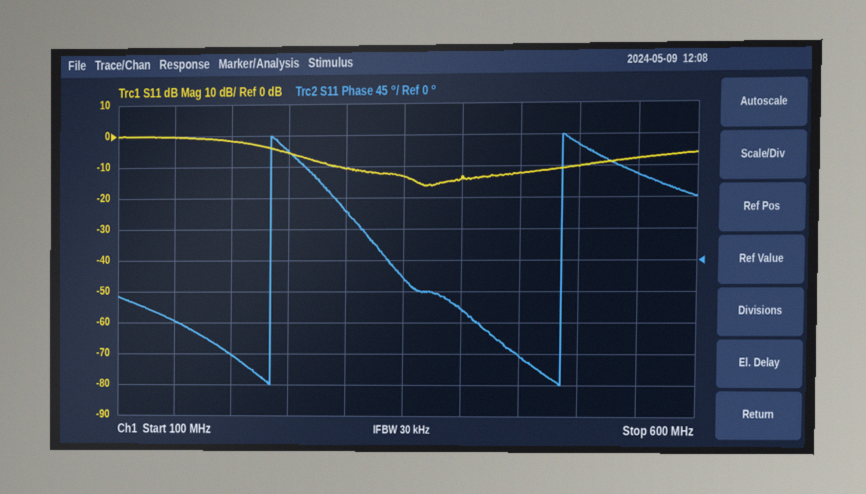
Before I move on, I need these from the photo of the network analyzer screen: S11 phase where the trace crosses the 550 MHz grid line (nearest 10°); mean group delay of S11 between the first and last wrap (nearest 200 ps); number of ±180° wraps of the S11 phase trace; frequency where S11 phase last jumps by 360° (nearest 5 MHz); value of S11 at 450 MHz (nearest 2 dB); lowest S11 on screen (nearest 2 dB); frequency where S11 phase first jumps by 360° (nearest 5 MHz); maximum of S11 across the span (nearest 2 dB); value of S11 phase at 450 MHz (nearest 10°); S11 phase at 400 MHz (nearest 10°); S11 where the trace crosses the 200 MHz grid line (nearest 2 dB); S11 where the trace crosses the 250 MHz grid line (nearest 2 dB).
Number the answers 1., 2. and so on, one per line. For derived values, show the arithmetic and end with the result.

1. 120°
2. 1 cycle / (485 MHz − 235 MHz) ≈ 4.0 ns
3. 2
4. 485 MHz
5. -12 dB
6. -16 dB
7. 235 MHz
8. 0 dB
9. -140°
10. -70°
11. -2 dB
12. -6 dB
